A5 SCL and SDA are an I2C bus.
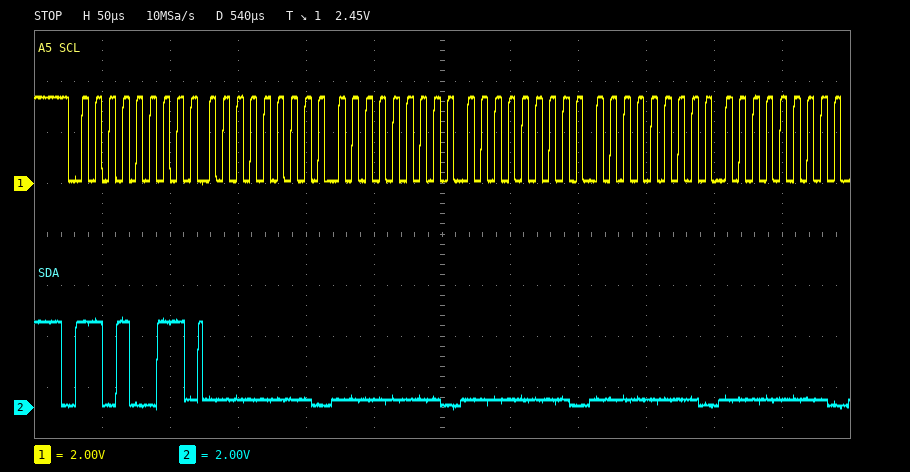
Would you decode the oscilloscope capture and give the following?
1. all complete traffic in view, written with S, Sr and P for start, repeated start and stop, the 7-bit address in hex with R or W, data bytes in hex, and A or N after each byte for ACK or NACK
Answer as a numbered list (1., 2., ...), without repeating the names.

1. S 69R A 00 A 00 A 00 A 00 A 00 A
